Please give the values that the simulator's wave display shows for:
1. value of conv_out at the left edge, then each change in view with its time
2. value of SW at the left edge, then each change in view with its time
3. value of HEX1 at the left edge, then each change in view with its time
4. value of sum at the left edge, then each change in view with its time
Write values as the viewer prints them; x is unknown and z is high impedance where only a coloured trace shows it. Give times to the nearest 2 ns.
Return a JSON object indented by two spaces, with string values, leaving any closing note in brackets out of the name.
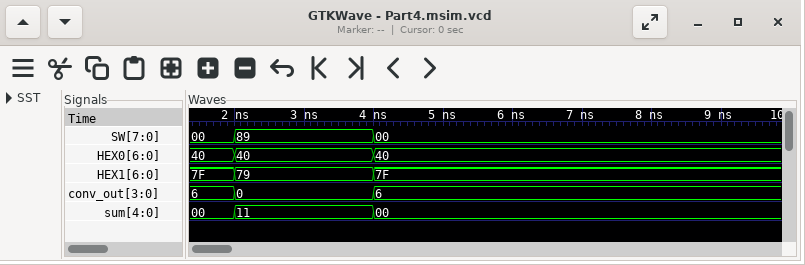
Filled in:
{
  "value of conv_out at the left edge, then each change in view with its time": "6, 0 at 2 ns, 6 at 4 ns",
  "value of SW at the left edge, then each change in view with its time": "00, 89 at 2 ns, 00 at 4 ns",
  "value of HEX1 at the left edge, then each change in view with its time": "7F, 79 at 2 ns, 7F at 4 ns",
  "value of sum at the left edge, then each change in view with its time": "00, 11 at 2 ns, 00 at 4 ns"
}
